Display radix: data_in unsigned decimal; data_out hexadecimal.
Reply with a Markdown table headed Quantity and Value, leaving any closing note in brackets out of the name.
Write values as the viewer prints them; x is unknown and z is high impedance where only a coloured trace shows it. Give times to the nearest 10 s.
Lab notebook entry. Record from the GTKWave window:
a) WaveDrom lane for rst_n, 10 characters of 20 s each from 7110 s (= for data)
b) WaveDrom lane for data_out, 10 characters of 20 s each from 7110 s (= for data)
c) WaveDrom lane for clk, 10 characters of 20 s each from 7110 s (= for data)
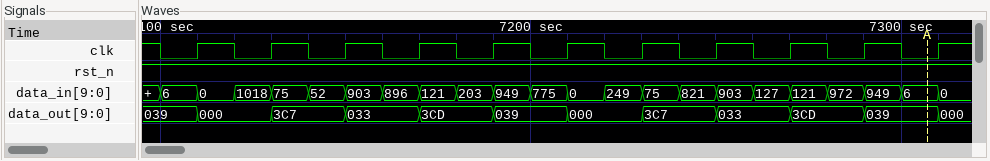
| Quantity | Value |
|---|---|
| WaveDrom lane for rst_n, 10 characters of 20 s each from 7110 s | {name: 'rst_n', wave: '1.........'} |
| WaveDrom lane for data_out, 10 characters of 20 s each from 7110 s | {name: 'data_out', wave: '==========', data: '000 3C7 033 3CD 039 000 3C7 033 3CD 039'} |
| WaveDrom lane for clk, 10 characters of 20 s each from 7110 s | {name: 'clk', wave: 'p.........'} |
